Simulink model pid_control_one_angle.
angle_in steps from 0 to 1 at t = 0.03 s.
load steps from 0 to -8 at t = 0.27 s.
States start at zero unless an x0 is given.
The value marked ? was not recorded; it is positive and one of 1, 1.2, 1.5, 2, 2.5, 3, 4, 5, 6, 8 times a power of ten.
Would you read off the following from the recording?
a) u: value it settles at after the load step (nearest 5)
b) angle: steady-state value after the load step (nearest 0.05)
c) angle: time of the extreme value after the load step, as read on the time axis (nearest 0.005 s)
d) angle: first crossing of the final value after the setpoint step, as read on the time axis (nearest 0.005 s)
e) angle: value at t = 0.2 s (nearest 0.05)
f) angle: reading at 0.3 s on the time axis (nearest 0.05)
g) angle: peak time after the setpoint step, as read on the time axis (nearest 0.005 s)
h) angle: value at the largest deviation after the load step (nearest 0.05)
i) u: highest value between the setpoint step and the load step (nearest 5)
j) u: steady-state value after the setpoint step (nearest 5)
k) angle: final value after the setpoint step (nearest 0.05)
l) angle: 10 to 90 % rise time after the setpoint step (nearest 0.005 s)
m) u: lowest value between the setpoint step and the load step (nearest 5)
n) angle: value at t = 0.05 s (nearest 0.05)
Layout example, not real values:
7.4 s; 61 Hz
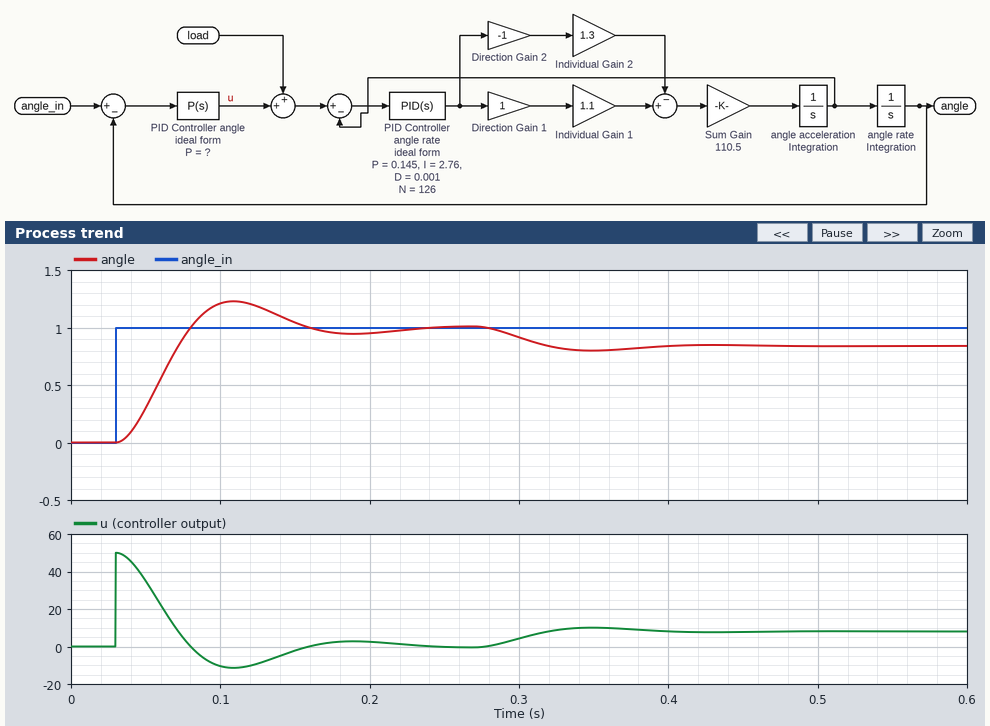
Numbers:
10; 0.85; 0.350 s; 0.080 s; 0.95; 0.90; 0.110 s; 0.80; 50; 0; 1.00; 0.035 s; -10; 0.30
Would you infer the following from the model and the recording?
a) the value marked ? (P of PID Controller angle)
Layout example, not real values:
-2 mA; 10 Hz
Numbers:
50
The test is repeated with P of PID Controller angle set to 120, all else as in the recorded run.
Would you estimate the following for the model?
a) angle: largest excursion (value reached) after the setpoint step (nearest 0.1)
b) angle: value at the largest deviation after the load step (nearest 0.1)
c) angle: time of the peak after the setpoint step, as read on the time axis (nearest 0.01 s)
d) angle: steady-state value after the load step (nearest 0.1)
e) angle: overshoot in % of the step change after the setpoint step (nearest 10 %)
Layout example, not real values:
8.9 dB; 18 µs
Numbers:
1.4; 0.9; 0.08 s; 0.9; 40 %
